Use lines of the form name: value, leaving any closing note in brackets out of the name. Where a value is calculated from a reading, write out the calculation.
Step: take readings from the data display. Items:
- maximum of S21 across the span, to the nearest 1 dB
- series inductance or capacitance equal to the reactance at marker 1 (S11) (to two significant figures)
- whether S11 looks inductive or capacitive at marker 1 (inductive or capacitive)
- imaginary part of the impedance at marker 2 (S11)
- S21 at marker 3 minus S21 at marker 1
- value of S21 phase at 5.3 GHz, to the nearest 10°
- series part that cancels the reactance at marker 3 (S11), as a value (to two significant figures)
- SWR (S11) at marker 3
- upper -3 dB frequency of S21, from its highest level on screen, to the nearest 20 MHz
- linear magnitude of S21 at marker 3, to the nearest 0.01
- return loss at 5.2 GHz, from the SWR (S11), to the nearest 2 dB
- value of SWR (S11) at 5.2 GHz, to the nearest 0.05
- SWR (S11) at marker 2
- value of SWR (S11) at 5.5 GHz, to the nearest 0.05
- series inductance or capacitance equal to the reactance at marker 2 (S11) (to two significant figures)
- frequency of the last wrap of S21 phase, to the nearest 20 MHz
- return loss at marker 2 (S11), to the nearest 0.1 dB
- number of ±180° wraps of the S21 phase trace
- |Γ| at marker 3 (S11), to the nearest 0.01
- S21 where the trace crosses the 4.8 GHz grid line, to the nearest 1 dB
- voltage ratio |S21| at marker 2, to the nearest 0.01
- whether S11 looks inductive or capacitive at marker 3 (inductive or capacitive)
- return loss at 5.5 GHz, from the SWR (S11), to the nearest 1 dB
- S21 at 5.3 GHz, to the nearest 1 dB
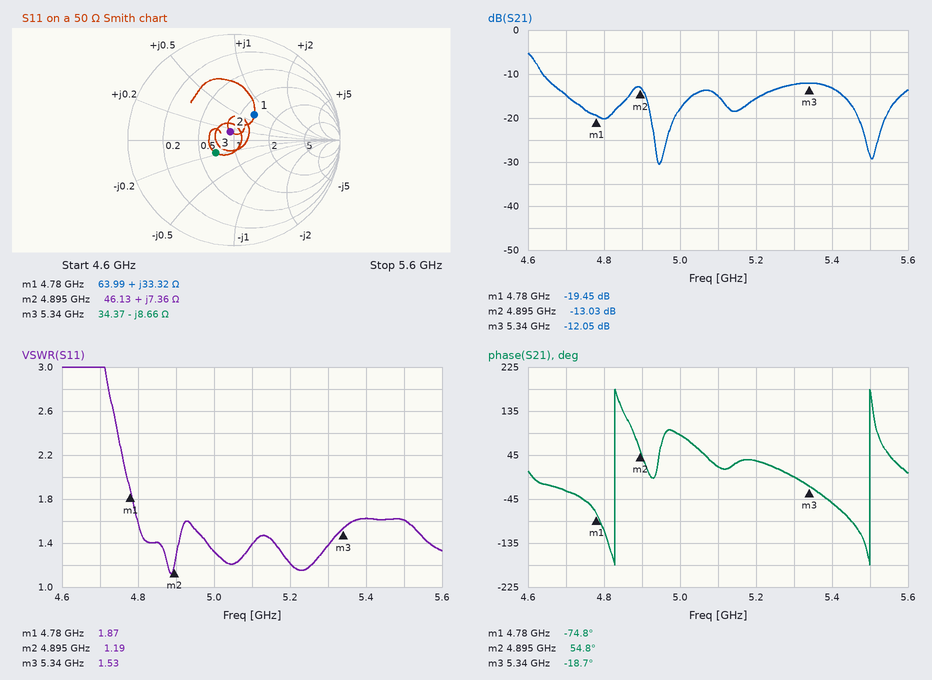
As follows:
maximum of S21 across the span, to the nearest 1 dB: -5 dB
series inductance or capacitance equal to the reactance at marker 1 (S11): L = 33.32 Ω/(2π × 4.78 GHz) ≈ 1.1 nH
whether S11 looks inductive or capacitive at marker 1: inductive
imaginary part of the impedance at marker 2: +7.36 Ω
S21 at marker 3 minus S21 at marker 1: -12.05 − (-19.45) = 7.40 dB
value of S21 phase at 5.3 GHz, to the nearest 10°: 0°
series part that cancels the reactance at marker 3 (S11), as a value: L = 8.66 Ω/(2π × 5.34 GHz) ≈ 258 pH, so 260 pH to two significant figures
SWR (S11) at marker 3: 1.53
upper -3 dB frequency of S21, from its highest level on screen, to the nearest 20 MHz: 4.62 GHz
linear magnitude of S21 at marker 3, to the nearest 0.01: 10^(-12.05/20) ≈ 0.25
return loss at 5.2 GHz, from the SWR (S11), to the nearest 2 dB: −20 log10((1.2 − 1)/(1.2 + 1)) ≈ 20.8 dB, so 20 dB to the nearest 2 dB
value of SWR (S11) at 5.2 GHz, to the nearest 0.05: 1.20
SWR (S11) at marker 2: 1.19
value of SWR (S11) at 5.5 GHz, to the nearest 0.05: 1.60
series inductance or capacitance equal to the reactance at marker 2 (S11): L = 7.36 Ω/(2π × 4.895 GHz) ≈ 239 pH, so 240 pH to two significant figures
frequency of the last wrap of S21 phase, to the nearest 20 MHz: 5.50 GHz
return loss at marker 2 (S11), to the nearest 0.1 dB: 21.3 dB
number of ±180° wraps of the S21 phase trace: 2
|Γ| at marker 3 (S11), to the nearest 0.01: 0.21
S21 where the trace crosses the 4.8 GHz grid line, to the nearest 1 dB: -20 dB
voltage ratio |S21| at marker 2, to the nearest 0.01: 10^(-13.03/20) ≈ 0.22
whether S11 looks inductive or capacitive at marker 3: capacitive
return loss at 5.5 GHz, from the SWR (S11), to the nearest 1 dB: −20 log10((1.6 − 1)/(1.6 + 1)) ≈ 13 dB
S21 at 5.3 GHz, to the nearest 1 dB: -12 dB
